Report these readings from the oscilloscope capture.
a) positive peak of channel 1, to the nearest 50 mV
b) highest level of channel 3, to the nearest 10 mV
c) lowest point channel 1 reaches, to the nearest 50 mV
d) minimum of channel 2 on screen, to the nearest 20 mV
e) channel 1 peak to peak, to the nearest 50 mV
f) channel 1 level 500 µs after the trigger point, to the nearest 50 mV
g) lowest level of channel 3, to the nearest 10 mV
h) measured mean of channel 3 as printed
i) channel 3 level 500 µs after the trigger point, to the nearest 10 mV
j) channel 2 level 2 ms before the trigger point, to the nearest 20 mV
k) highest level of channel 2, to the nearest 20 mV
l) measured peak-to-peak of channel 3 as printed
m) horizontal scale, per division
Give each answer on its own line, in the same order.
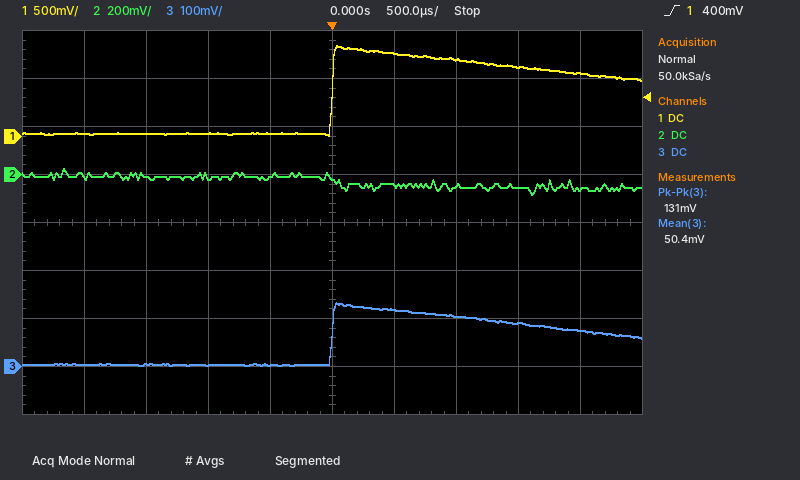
950 mV
130 mV
0 mV
-80 mV
950 mV
850 mV
0 mV
50.4 mV
120 mV
0 mV
20 mV
131 mV
500 µs
